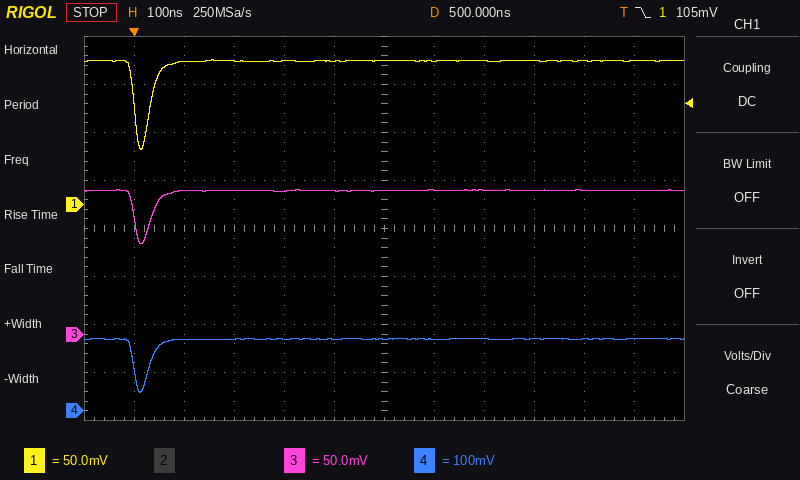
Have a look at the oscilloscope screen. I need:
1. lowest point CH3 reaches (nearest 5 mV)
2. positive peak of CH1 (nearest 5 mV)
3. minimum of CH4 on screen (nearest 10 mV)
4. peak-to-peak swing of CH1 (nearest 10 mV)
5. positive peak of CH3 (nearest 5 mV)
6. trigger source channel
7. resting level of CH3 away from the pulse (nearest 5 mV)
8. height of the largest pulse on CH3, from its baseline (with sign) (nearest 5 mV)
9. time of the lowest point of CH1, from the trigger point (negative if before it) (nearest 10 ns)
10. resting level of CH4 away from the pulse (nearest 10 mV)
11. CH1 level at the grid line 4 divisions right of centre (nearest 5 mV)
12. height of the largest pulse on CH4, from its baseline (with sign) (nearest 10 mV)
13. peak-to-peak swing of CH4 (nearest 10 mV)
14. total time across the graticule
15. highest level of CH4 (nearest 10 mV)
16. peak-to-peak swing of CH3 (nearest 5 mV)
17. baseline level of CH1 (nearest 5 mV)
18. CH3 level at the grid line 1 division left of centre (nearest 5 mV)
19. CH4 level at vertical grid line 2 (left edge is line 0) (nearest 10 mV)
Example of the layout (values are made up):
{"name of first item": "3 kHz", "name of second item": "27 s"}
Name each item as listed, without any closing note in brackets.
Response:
{"lowest point CH3 reaches": "95 mV", "positive peak of CH1": "150 mV", "minimum of CH4 on screen": "40 mV", "peak-to-peak swing of CH1": "90 mV", "positive peak of CH3": "150 mV", "trigger source channel": "CH1", "resting level of CH3 away from the pulse": "150 mV", "height of the largest pulse on CH3, from its baseline (with sign)": "-55 mV", "time of the lowest point of CH1, from the trigger point (negative if before it)": "+10 ns", "resting level of CH4 away from the pulse": "150 mV", "CH1 level at the grid line 4 divisions right of centre": "150 mV", "height of the largest pulse on CH4, from its baseline (with sign)": "-110 mV", "peak-to-peak swing of CH4": "110 mV", "total time across the graticule": "1.2 µs", "highest level of CH4": "150 mV", "peak-to-peak swing of CH3": "55 mV", "baseline level of CH1": "150 mV", "CH3 level at the grid line 1 division left of centre": "150 mV", "CH4 level at vertical grid line 2 (left edge is line 0)": "150 mV"}
